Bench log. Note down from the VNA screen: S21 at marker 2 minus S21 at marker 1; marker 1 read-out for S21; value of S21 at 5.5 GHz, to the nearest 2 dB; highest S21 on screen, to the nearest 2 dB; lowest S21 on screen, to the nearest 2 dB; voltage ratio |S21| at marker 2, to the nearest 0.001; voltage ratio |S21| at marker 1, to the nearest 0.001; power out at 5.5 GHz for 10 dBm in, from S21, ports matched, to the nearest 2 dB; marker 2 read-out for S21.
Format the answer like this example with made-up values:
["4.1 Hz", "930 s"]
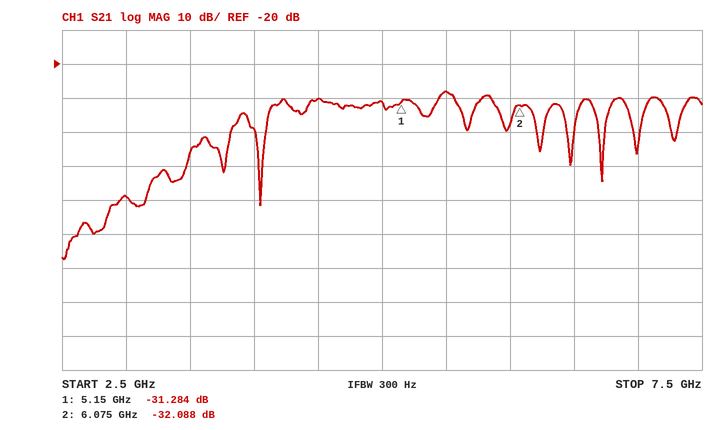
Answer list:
["-0.804 dB", "-31.284 dB", "-28 dB", "-28 dB", "-78 dB", "0.025", "0.027", "-18 dBm", "-32.088 dB"]
